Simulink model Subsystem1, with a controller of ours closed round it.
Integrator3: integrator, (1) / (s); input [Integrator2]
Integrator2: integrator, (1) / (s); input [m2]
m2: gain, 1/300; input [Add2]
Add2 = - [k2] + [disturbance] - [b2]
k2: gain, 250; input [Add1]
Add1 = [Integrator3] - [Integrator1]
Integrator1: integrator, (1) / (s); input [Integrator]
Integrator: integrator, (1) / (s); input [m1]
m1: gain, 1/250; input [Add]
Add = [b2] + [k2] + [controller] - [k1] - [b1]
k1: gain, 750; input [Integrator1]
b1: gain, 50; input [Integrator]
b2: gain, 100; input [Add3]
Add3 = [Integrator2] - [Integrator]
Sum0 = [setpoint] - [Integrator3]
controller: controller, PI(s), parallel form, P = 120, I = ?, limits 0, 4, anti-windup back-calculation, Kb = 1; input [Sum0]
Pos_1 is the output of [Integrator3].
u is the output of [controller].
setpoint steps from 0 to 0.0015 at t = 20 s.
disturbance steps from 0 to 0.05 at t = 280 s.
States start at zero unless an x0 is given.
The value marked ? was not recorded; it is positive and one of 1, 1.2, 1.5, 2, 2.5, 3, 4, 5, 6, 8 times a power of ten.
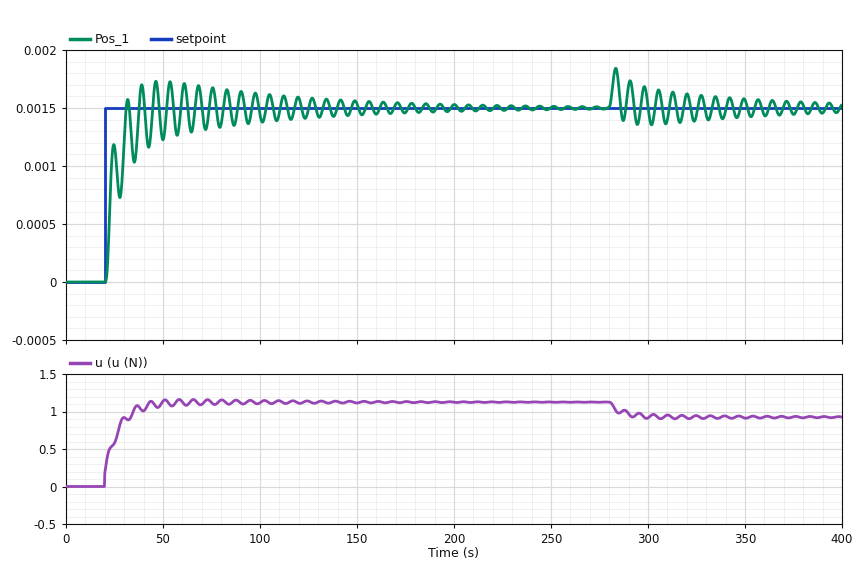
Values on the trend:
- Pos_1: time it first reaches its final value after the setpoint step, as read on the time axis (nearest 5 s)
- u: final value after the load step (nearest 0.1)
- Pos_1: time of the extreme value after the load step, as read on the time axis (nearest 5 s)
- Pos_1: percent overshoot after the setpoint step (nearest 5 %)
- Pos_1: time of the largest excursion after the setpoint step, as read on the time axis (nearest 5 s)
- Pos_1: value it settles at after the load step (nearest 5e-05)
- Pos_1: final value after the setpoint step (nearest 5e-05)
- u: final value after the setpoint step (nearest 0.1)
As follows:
30 s
0.9
285 s
15 %
45 s
0.00150
0.00150
1.1
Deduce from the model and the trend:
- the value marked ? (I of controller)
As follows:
120
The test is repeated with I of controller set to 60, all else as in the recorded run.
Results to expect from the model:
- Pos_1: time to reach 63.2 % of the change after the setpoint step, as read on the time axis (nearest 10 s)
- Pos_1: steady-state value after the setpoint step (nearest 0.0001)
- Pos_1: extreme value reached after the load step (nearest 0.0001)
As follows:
30 s
0.0015
0.0019
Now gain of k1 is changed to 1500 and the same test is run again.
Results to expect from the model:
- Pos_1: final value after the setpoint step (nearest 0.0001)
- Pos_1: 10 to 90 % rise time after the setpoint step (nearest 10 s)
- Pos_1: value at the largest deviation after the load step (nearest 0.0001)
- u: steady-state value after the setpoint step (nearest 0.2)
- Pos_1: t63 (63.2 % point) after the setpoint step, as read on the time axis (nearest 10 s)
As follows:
0.0015
30 s
0.0018
2.2
30 s
